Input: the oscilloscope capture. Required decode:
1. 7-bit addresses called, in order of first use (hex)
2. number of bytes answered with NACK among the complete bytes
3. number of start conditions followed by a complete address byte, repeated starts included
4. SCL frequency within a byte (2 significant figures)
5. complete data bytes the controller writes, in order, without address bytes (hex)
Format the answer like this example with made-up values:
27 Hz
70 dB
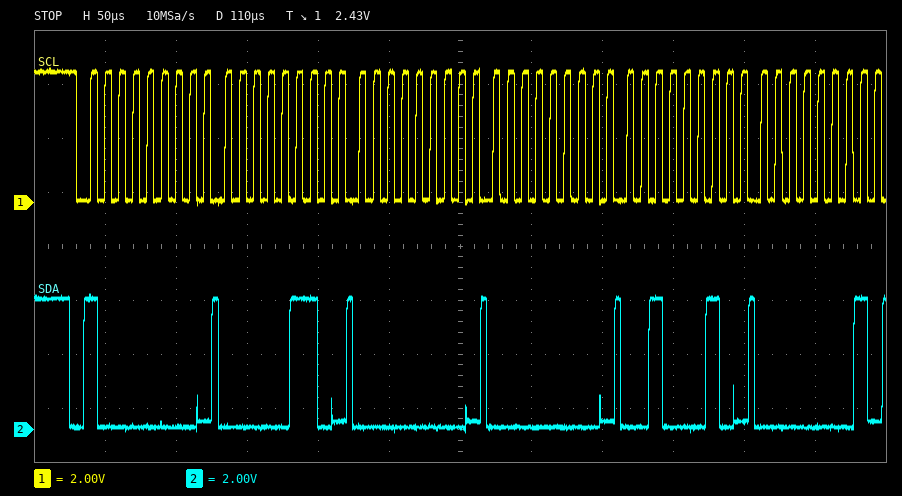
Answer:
0x40
0
1
100 kHz
06 00 00 22 01
